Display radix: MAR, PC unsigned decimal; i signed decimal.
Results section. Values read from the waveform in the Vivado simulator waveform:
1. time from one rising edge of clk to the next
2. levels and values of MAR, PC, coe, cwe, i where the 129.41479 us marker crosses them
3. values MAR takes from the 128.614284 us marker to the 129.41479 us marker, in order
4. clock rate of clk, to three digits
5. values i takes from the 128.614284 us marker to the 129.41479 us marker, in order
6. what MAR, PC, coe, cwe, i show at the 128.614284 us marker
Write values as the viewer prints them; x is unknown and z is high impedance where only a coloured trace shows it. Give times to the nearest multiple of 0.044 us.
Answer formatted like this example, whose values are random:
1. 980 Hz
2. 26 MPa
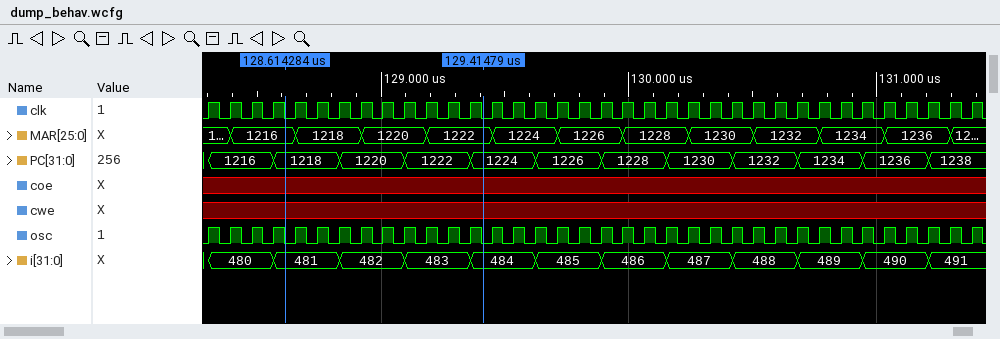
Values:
1. 0.088 us
2. MAR=1222, PC=1224, coe=x, cwe=x, i=484
3. 1216, 1218, 1220, 1222
4. 11.4 MHz
5. 481, 482, 483, 484
6. MAR=1216, PC=1218, coe=x, cwe=x, i=481
